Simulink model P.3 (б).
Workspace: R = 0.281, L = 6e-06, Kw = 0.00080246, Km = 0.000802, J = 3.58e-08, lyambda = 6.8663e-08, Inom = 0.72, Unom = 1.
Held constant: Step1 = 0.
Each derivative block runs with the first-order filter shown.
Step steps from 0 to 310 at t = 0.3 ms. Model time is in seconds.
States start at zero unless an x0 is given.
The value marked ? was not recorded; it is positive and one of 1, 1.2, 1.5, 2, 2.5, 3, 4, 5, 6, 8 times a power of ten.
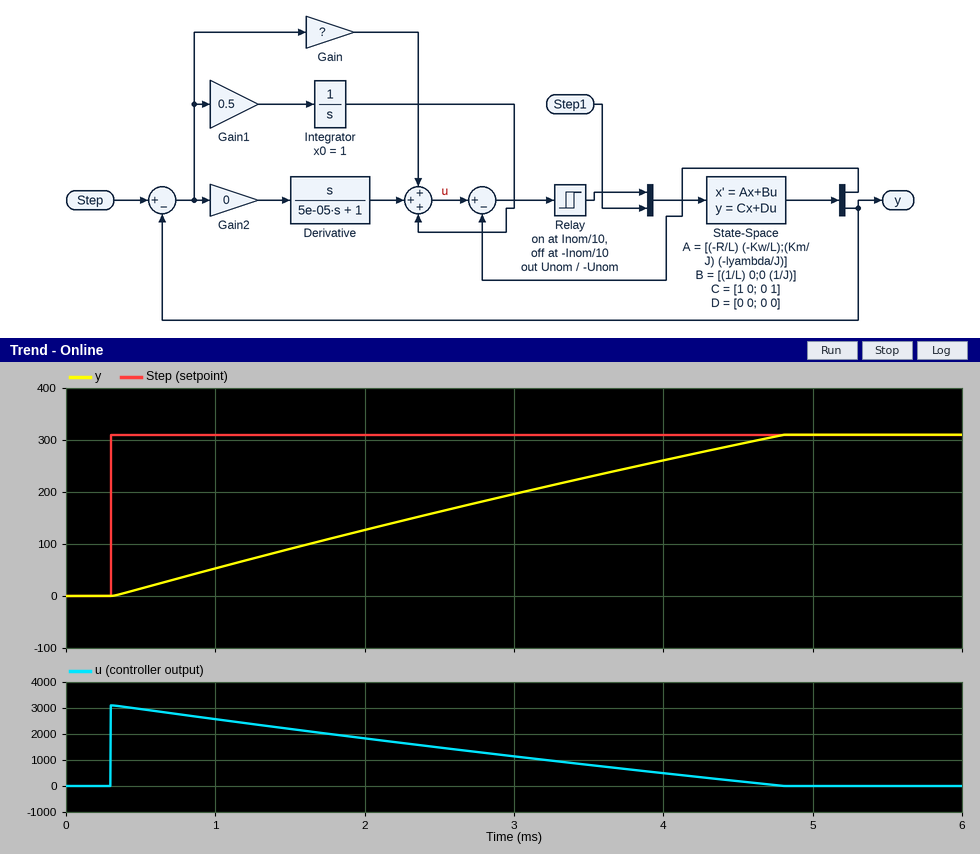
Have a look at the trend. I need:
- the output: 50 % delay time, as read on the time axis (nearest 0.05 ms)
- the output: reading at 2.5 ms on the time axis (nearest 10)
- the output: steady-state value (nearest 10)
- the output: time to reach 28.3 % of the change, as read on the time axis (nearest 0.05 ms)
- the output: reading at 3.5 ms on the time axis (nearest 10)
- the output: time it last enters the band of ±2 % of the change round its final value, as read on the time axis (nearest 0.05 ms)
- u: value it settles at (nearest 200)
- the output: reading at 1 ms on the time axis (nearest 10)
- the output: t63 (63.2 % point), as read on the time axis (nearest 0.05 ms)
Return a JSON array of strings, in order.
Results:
["2.40 ms", "160", "310", "1.45 ms", "230", "4.70 ms", "0", "50", "3.00 ms"]
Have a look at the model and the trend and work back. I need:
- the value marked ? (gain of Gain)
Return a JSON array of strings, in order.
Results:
["10"]
